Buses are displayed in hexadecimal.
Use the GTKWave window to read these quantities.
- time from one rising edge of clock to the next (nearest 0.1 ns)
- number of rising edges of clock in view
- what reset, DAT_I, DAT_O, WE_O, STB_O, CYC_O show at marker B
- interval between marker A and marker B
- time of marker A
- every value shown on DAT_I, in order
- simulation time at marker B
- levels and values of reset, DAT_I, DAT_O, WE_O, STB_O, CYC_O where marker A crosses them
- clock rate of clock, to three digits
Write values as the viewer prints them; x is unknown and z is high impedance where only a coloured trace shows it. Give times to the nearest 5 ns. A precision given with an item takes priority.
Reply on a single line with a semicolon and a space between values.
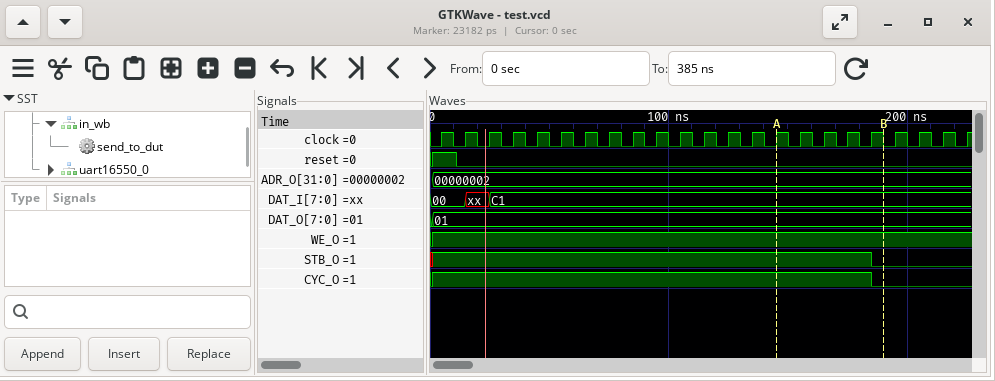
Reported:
10 ns; 23; reset=0, DAT_I=C1, DAT_O=01, WE_O=1, STB_O=0, CYC_O=0; 45 ns; 145 ns; 00, xx, C1; 190 ns; reset=0, DAT_I=C1, DAT_O=01, WE_O=1, STB_O=1, CYC_O=1; 100 MHz
